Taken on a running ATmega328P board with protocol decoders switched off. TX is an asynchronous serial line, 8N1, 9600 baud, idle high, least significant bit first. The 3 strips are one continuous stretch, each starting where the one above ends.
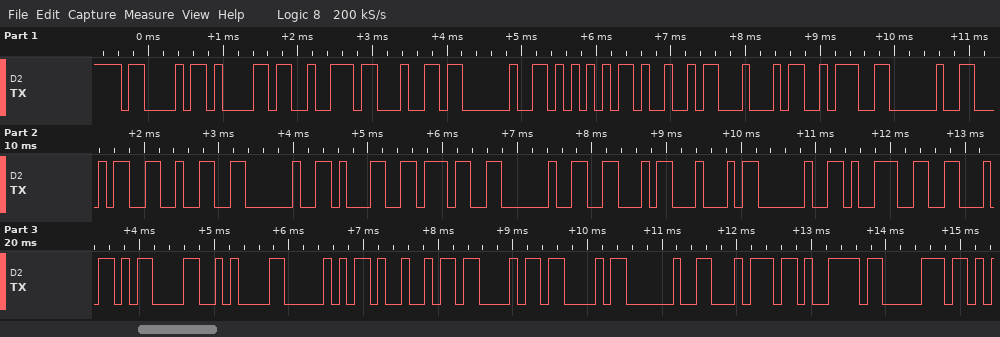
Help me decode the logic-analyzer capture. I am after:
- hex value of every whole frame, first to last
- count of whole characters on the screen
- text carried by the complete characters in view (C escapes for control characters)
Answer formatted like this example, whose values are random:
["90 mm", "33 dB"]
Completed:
["43 61 72 64 20 55 49 44 3A 20 34 32 20 31 37 20 46 44 20 39 46 0D 0A 50 49 43 43 20 74 79 70", "31", "\"Card UID: 42 17 FD 9F\\r\\nPICC typ\""]
